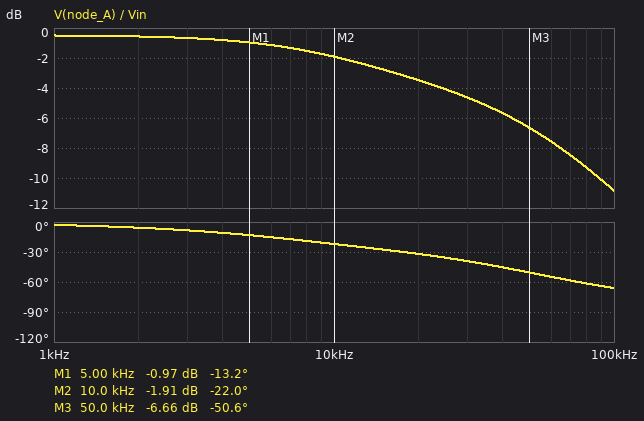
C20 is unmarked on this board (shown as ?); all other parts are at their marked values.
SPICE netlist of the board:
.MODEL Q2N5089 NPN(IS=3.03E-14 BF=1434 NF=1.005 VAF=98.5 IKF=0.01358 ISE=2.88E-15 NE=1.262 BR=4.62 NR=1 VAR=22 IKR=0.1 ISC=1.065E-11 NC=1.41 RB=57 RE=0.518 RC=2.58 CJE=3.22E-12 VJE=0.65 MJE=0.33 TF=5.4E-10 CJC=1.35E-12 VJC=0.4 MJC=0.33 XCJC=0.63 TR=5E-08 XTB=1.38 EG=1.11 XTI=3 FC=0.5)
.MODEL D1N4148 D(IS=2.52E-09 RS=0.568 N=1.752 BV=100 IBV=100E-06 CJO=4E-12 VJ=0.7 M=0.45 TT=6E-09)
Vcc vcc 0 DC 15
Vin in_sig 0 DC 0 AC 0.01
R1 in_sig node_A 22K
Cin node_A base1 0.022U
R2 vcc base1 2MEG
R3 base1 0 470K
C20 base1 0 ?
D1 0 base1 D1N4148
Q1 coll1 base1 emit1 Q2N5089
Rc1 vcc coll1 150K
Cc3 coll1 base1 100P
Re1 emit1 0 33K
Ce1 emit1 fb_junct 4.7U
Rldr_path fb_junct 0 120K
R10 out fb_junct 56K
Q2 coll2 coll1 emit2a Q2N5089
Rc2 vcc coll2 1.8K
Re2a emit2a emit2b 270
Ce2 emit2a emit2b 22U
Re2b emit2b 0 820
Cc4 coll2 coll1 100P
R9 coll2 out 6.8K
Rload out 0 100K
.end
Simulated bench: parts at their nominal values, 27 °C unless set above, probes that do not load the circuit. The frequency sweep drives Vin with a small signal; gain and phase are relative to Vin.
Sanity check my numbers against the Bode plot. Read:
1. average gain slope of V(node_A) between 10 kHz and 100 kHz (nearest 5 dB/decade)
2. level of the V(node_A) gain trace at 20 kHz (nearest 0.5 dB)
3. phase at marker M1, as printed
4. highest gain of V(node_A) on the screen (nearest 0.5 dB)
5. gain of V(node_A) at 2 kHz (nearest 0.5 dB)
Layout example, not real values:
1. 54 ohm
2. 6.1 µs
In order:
1. -10 dB/decade
2. -3.5 dB
3. -13.2 deg
4. -0.5 dB
5. -0.5 dB
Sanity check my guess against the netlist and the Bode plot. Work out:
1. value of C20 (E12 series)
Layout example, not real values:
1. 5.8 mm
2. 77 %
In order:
1. 150 pF
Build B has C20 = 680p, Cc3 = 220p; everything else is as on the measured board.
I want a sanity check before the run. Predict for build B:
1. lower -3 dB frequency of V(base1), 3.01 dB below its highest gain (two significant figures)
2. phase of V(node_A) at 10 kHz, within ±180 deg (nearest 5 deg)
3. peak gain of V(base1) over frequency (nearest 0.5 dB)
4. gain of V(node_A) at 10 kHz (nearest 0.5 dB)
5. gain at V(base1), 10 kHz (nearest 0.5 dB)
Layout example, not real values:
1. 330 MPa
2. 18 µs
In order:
1. 17 Hz
2. -45 deg
3. -1.0 dB
4. -5.5 dB
5. -6.0 dB
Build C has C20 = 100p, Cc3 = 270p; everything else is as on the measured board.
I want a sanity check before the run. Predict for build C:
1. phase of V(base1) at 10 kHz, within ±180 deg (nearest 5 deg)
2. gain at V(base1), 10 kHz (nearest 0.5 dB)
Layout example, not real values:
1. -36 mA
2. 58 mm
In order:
1. -25 deg
2. -4.0 dB
